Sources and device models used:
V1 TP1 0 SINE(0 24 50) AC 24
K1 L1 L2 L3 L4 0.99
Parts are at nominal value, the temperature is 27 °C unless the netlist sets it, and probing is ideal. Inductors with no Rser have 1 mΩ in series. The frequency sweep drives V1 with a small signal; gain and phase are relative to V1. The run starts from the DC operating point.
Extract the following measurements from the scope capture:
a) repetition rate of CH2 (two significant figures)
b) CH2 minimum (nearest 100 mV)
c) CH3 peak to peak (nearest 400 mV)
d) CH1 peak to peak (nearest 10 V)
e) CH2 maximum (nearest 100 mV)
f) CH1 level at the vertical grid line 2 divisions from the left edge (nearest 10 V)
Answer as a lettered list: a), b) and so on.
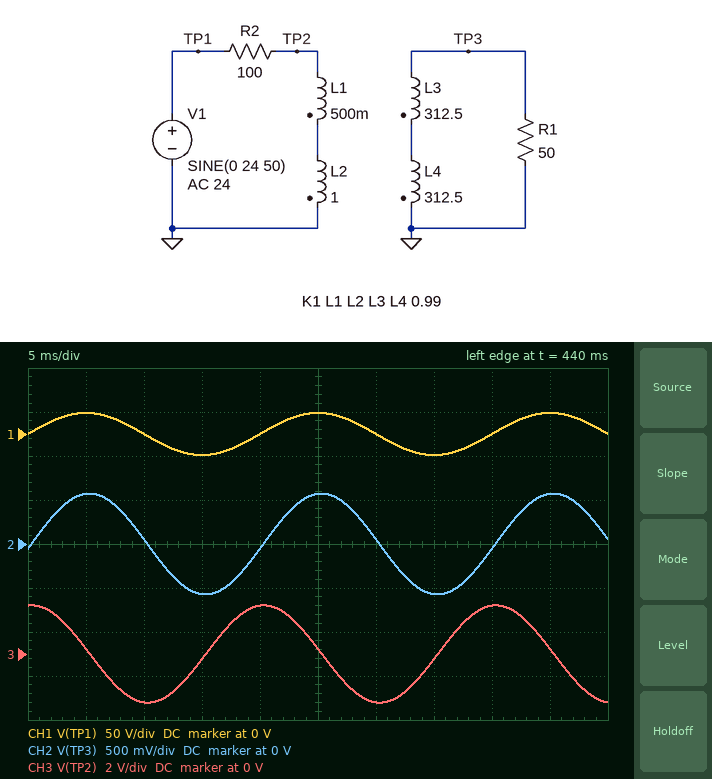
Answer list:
a) 50 Hz
b) -600 mV
c) 4.4 V
d) 50 V
e) 600 mV
f) 0 V
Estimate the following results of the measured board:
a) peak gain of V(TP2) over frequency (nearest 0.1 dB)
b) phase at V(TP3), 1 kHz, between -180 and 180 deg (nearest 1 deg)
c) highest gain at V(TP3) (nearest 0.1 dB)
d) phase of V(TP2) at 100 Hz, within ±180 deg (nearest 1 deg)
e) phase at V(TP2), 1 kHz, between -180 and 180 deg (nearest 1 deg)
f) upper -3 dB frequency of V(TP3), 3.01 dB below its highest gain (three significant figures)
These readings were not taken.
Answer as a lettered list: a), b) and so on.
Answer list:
a) 0 dB
b) -62 deg
c) -32.4 dB
d) 79 deg
e) 28 deg
f) 540 Hz
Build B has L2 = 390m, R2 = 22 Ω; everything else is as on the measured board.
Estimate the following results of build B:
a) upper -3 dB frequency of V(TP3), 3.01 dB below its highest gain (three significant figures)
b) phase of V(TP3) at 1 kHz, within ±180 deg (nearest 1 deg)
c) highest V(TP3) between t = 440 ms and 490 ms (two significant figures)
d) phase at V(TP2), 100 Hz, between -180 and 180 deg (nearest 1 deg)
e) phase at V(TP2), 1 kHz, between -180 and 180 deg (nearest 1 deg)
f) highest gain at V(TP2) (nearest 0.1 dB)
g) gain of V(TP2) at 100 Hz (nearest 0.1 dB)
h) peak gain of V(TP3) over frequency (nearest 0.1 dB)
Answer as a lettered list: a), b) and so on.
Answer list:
a) 198 Hz
b) -79 deg
c) 2.0 V
d) 63 deg
e) 11 deg
f) 0 dB
g) -6.9 dB
h) -21.4 dB
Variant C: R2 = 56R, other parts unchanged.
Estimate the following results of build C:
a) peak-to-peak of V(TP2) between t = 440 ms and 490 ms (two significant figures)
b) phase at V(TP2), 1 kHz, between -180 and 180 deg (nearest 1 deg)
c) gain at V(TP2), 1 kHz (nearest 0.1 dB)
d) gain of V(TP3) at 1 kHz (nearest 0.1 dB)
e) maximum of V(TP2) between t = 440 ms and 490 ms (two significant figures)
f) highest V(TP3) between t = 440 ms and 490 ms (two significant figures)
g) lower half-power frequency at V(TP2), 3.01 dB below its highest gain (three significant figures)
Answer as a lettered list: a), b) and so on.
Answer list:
a) 7.8 V
b) 17 deg
c) -0.4 dB
d) -38.1 dB
e) 3.9 V
f) 1.0 V
g) 303 Hz
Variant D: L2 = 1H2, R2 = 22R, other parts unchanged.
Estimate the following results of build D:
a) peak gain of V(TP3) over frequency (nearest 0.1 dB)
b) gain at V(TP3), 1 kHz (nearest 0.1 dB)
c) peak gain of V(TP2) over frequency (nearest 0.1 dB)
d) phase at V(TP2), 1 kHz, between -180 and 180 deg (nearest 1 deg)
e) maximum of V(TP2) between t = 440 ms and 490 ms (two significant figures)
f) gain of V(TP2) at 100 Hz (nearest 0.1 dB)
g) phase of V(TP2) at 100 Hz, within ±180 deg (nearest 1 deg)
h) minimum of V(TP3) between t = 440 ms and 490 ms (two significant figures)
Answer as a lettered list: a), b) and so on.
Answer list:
a) -18.8 dB
b) -38.3 dB
c) 0 dB
d) 6 deg
e) 10 V
f) -3.3 dB
g) 46 deg
h) -2.5 V
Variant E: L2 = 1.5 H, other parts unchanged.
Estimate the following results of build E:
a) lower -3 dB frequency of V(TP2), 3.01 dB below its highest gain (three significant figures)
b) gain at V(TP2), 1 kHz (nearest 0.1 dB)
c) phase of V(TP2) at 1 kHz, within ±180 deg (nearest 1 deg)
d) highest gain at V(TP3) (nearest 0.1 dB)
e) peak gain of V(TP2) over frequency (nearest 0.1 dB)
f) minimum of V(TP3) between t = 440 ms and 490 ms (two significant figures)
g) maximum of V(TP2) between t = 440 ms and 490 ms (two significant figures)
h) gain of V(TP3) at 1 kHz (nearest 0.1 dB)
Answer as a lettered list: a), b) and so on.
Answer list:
a) 413 Hz
b) -0.7 dB
c) 22 deg
d) -31.3 dB
e) 0 dB
f) -650 mV
g) 2.9 V
h) -39.7 dB
